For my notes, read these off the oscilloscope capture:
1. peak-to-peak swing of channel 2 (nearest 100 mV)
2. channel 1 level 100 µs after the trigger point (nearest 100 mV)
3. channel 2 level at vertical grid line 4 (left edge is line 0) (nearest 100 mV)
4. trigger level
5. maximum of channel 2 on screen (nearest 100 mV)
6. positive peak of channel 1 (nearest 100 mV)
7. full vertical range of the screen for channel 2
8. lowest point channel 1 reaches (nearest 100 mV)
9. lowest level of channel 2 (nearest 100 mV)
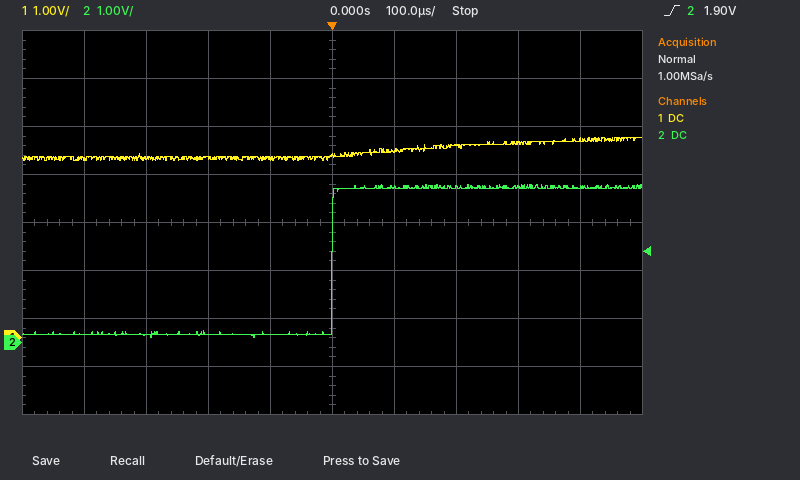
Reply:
3.2 V
3.9 V
200 mV
1.90 V
3.3 V
4.2 V
8 V
3.7 V
100 mV
